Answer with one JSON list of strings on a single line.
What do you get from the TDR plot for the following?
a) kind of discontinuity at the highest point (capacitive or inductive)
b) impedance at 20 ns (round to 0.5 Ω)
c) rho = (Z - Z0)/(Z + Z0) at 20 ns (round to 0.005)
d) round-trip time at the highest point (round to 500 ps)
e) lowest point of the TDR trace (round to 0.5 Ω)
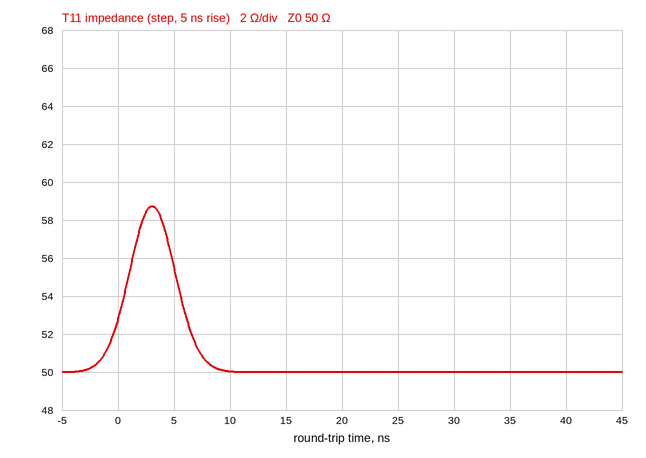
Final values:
["inductive", "50.0 Ω", "0.000", "3.0 ns", "50.0 Ω"]
